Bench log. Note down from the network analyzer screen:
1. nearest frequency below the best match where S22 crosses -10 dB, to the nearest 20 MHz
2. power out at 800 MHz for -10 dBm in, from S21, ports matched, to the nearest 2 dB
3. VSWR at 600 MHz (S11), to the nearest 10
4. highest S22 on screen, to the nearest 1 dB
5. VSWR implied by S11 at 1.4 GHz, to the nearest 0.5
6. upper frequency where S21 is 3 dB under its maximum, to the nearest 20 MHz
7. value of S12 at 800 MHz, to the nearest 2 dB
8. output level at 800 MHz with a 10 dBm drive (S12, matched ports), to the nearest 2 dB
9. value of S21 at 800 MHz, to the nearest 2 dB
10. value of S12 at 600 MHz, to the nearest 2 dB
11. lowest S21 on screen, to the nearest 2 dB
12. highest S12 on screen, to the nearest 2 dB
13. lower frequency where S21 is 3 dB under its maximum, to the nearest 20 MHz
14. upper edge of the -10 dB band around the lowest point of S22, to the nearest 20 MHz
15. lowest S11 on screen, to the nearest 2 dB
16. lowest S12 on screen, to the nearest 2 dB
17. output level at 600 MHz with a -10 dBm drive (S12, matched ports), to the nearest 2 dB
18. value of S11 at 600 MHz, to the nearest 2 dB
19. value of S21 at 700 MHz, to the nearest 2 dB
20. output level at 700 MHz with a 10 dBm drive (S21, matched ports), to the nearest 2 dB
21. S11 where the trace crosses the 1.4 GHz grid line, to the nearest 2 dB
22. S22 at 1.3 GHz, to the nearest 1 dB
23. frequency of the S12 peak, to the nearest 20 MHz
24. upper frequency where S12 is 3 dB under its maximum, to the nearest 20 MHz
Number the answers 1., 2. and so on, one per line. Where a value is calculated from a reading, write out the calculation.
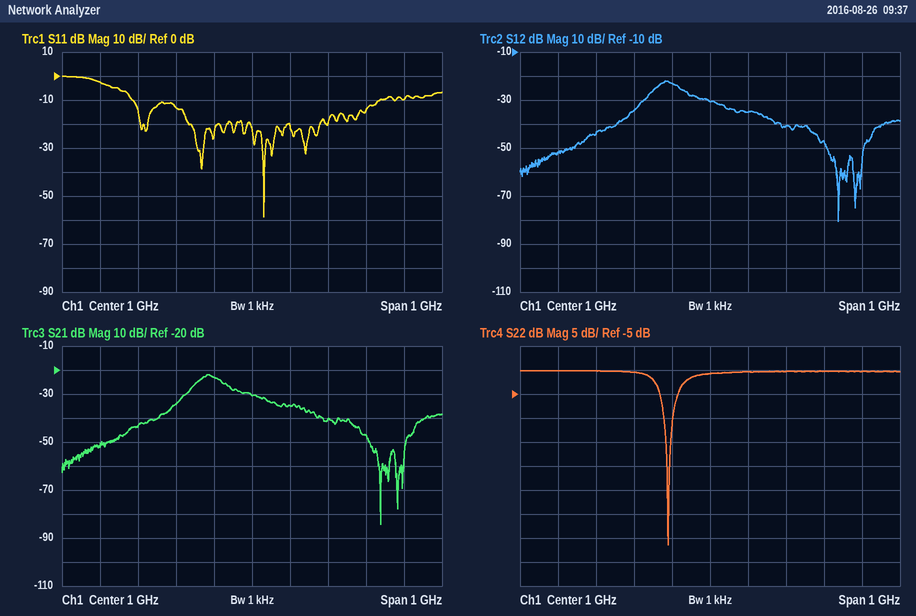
1. 880 MHz
2. -10 dBm + (-34 dB) = -44 dBm
3. |Γ| = 10^(-2/20) = 0.7943; VSWR = (1 + 0.7943)/(1 − 0.7943) ≈ 8.72, so 10 to the nearest 10
4. 0 dB
5. |Γ| = 10^(-10/20) = 0.3162; VSWR = (1 + 0.3162)/(1 − 0.3162) ≈ 1.92, so 2.0 to the nearest 0.5
6. 920 MHz
7. -34 dB
8. 10 dBm + (-34 dB) = -24 dBm
9. -34 dB
10. -52 dB
11. -84 dB
12. -22 dB
13. 860 MHz
14. 900 MHz
15. -58 dB
16. -80 dB
17. -10 dBm + (-52 dB) = -62 dBm
18. -2 dB
19. -44 dB
20. 10 dBm + (-44 dB) = -34 dBm
21. -10 dB
22. 0 dB
23. 880 MHz
24. 920 MHz
